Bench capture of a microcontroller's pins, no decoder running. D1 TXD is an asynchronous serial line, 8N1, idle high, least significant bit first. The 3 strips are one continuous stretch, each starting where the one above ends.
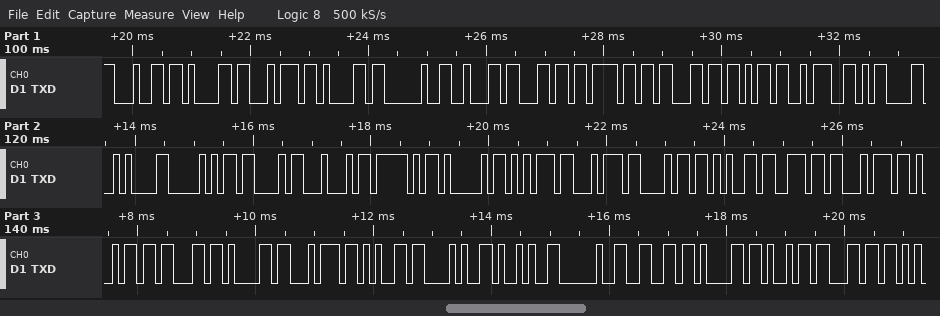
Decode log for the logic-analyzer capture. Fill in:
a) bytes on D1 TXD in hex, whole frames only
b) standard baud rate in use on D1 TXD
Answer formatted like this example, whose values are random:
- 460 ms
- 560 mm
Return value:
- 64 61 74 61 20 62 6C 6F 63 6B 3A 0D 0A 50 43 44 5F 41 75 74 68 65 6E 74 69 63 61 74 65 28 29 20 66 61 69 6C
- 9600 baud
